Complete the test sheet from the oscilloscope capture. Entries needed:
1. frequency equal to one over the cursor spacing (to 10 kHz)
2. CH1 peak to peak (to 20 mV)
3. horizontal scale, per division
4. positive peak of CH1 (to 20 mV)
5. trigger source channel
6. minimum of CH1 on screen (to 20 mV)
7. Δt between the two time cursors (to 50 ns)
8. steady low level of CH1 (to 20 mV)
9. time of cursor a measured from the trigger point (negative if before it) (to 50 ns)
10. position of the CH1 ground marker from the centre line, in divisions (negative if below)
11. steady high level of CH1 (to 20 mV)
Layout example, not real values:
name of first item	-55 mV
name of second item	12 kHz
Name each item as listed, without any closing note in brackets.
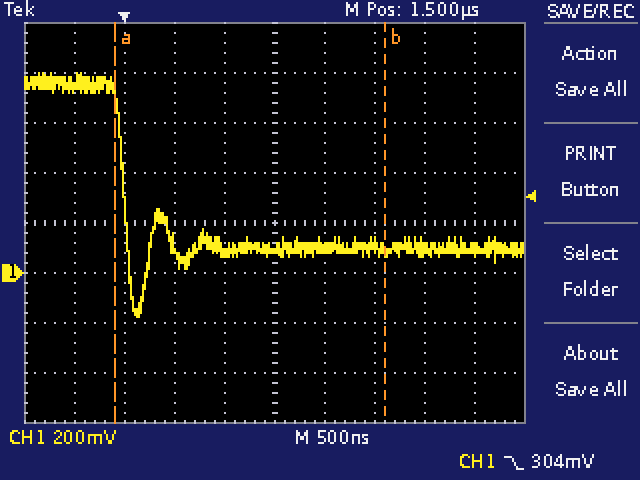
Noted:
frequency equal to one over the cursor spacing	370 kHz
CH1 peak to peak	980 mV
horizontal scale, per division	500 ns
positive peak of CH1	800 mV
trigger source channel	CH1
minimum of CH1 on screen	-180 mV
Δt between the two time cursors	2.70 µs
steady low level of CH1	100 mV
time of cursor a measured from the trigger point (negative if before it)	-100 ns
position of the CH1 ground marker from the centre line, in divisions	-1.0 div
steady high level of CH1	760 mV
